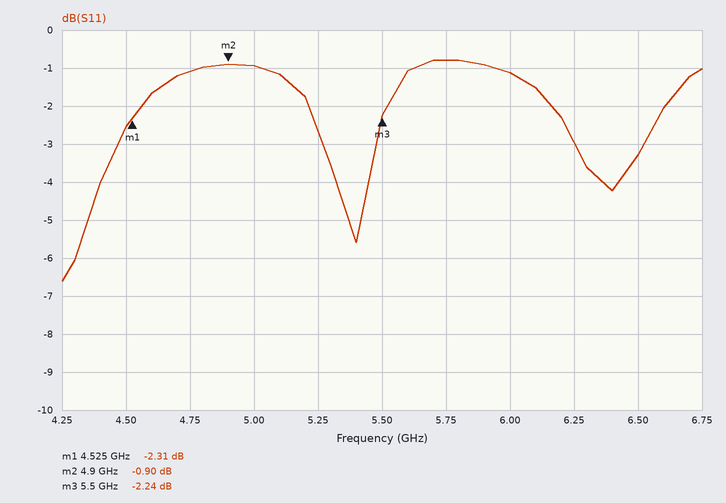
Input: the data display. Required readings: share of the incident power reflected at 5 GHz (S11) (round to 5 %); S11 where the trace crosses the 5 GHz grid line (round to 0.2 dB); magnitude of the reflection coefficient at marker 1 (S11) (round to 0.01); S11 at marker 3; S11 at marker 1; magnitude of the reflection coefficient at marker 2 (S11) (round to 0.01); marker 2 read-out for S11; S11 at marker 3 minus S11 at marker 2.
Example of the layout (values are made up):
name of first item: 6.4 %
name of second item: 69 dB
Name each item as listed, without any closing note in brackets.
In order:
share of the incident power reflected at 5 GHz (S11): 80 %
S11 where the trace crosses the 5 GHz grid line: -1.0 dB
magnitude of the reflection coefficient at marker 1 (S11): 0.77
S11 at marker 3: -2.24 dB
S11 at marker 1: -2.31 dB
magnitude of the reflection coefficient at marker 2 (S11): 0.90
marker 2 read-out for S11: -0.90 dB
S11 at marker 3 minus S11 at marker 2: -1.34 dB
